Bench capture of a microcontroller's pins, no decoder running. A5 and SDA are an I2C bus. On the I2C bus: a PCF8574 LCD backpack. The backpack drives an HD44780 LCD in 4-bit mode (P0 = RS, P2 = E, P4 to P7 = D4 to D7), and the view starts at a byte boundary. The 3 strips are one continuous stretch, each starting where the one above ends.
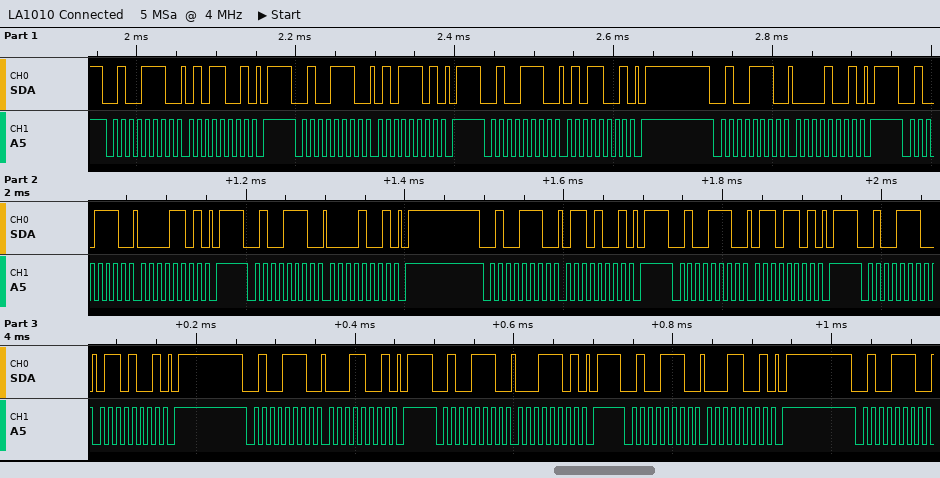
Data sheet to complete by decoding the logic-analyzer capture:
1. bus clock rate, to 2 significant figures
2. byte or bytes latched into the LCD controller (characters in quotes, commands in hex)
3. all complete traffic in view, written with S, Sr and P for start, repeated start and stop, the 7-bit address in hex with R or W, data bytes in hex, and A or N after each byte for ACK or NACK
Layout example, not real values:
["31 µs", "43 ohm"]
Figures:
["100 kHz", "'P' 'a'", "S 27W A 59 A P S 27W A 5D A P S 27W A 59 A P S 27W A 09 A P S 27W A 0D A P S 27W A 09 A P S 27W A 69 A P S 27W A 6D A P S 27W A 69 A P S 27W A 19 A P S 27W A 1D A P S 27W A 19 A P S 27W A"]
